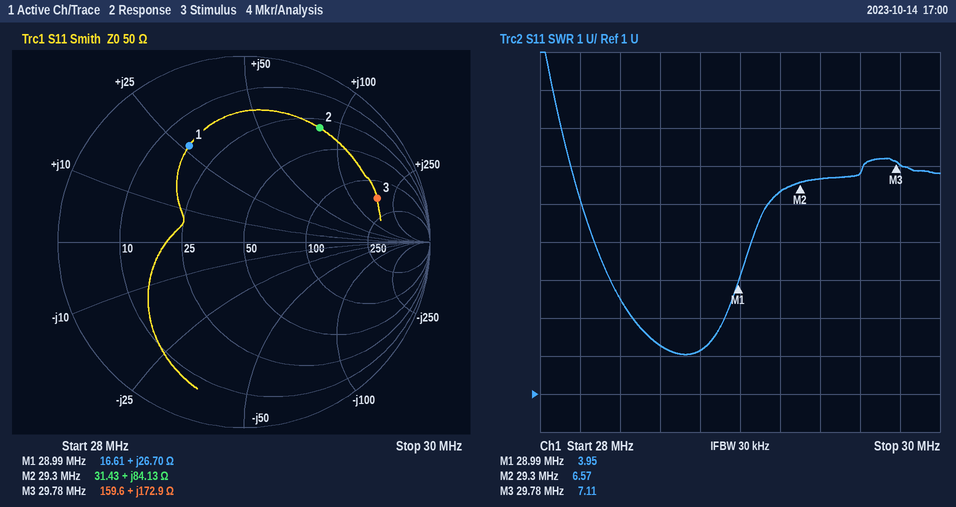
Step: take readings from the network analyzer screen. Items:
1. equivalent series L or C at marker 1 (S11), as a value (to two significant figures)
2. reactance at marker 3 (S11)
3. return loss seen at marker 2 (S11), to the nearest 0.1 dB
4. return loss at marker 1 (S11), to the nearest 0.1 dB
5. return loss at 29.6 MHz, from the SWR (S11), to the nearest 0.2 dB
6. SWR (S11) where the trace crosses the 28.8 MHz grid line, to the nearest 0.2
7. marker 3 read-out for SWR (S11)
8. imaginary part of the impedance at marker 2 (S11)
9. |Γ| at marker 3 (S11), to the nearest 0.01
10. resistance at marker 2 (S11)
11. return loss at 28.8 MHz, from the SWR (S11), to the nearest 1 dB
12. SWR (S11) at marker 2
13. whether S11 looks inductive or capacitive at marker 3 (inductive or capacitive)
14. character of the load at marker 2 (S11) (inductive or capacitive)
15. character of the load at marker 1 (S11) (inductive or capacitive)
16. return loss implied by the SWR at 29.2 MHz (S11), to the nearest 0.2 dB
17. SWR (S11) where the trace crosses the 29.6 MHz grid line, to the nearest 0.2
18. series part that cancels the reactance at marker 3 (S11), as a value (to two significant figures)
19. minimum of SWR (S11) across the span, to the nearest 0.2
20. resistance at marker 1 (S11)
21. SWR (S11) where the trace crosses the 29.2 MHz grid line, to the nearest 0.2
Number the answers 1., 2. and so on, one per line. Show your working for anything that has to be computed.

1. L = 26.7 Ω/(2π × 28.99 MHz) ≈ 147 nH, so 150 nH to two significant figures
2. +172.9 Ω
3. 2.7 dB
4. 4.5 dB
5. −20 log10((6.8 − 1)/(6.8 + 1)) ≈ 2.6 dB
6. 2.2
7. 7.11
8. +84.13 Ω
9. 0.75
10. 31.43 Ω
11. −20 log10((2.2 − 1)/(2.2 + 1)) ≈ 9 dB
12. 6.57
13. inductive
14. inductive
15. inductive
16. −20 log10((6.4 − 1)/(6.4 + 1)) ≈ 2.74 dB, so 2.8 dB to the nearest 0.2 dB
17. 6.8
18. C = 1/(2π × 29.78 MHz × 172.9 Ω) ≈ 31 pF
19. 2.0
20. 16.61 Ω
21. 6.4
